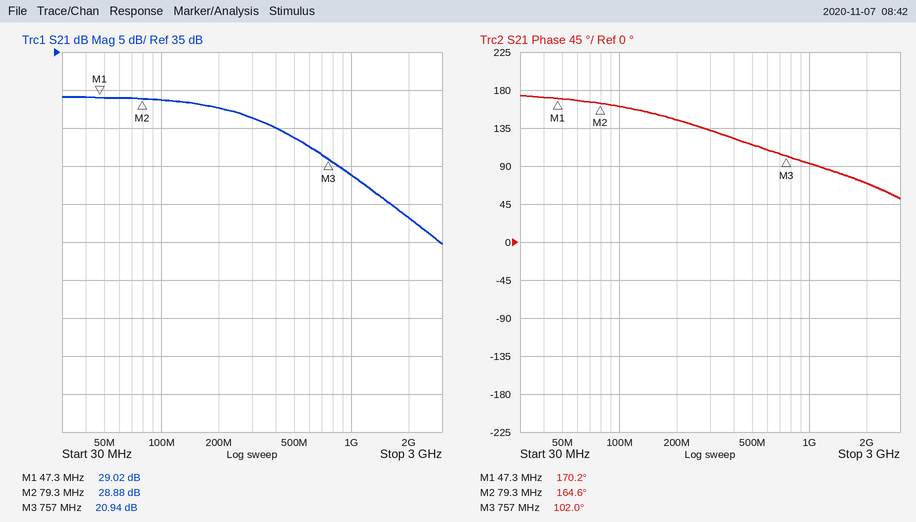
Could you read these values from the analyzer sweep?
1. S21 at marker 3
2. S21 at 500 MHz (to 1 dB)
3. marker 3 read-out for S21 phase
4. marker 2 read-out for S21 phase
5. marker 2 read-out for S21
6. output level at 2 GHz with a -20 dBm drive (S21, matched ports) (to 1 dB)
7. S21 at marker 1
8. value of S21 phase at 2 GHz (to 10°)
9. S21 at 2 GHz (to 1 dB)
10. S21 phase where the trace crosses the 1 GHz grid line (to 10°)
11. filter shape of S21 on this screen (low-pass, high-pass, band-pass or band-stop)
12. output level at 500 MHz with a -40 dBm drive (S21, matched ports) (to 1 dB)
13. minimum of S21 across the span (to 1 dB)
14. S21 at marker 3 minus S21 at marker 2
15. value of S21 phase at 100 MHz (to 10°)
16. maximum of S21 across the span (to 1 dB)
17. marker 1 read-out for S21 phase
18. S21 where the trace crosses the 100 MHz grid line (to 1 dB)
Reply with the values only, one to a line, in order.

20.94 dB
24 dB
102.0°
164.6°
28.88 dB
-7 dBm
29.02 dB
70°
13 dB
90°
low-pass
-16 dBm
10 dB
-7.94 dB
160°
29 dB
170.2°
29 dB
